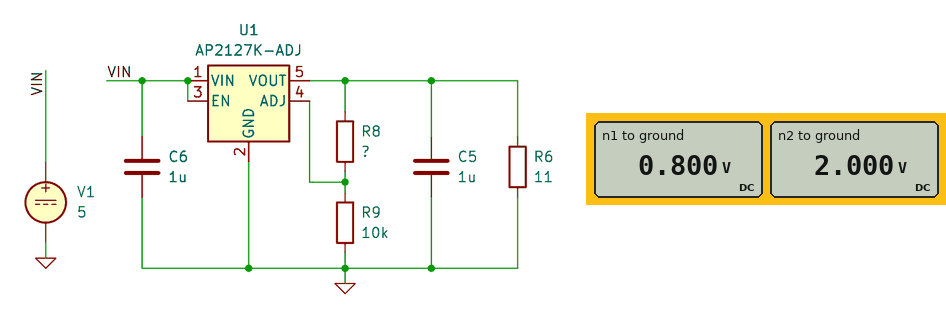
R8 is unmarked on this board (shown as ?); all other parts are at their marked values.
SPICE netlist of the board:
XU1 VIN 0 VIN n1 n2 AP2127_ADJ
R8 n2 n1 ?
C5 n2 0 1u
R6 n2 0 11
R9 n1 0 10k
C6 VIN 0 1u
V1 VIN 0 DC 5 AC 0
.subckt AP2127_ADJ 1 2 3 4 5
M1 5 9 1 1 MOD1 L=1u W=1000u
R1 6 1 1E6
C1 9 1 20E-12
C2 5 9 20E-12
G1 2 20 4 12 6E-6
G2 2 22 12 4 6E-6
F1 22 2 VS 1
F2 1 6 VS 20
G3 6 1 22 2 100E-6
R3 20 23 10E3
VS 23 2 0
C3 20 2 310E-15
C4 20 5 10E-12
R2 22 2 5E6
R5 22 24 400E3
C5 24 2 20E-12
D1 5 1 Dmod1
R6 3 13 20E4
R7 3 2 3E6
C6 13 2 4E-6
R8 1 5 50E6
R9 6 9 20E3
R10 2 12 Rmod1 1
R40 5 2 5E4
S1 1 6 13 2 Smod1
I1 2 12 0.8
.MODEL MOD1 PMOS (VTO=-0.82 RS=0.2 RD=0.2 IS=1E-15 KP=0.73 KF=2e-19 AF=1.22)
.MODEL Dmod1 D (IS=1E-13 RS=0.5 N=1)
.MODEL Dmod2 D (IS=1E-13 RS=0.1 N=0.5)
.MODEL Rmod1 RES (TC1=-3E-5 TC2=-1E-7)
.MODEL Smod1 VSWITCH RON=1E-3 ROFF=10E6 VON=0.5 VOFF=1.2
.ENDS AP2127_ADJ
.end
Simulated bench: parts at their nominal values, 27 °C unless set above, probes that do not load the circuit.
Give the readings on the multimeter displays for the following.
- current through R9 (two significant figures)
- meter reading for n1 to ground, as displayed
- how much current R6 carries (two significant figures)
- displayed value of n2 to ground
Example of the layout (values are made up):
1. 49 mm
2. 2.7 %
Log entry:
1. 80 µA
2. 0.800 V
3. 180 mA
4. 2.000 V
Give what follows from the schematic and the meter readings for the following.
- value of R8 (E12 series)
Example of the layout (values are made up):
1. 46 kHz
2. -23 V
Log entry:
1. 15 kΩ
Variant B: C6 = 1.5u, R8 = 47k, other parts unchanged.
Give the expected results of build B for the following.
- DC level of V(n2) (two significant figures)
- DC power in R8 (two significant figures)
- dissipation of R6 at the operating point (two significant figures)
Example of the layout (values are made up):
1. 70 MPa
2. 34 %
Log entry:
1. 4.6 V
2. 300 µW
3. 1.9 W
